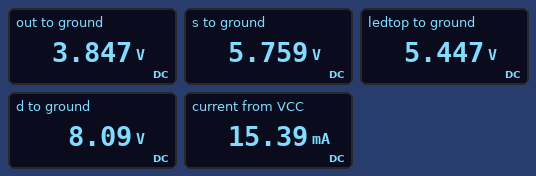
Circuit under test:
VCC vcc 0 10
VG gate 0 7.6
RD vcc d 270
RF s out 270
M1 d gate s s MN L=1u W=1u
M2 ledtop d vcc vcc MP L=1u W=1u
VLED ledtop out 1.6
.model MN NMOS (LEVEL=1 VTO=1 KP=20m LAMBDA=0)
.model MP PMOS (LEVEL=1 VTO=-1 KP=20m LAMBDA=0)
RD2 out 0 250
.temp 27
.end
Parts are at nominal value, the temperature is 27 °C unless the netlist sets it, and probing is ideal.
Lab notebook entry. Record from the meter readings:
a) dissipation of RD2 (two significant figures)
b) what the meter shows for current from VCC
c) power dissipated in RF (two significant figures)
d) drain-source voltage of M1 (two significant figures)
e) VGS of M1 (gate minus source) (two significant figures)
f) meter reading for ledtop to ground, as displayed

59 mW
15.39 mA
14 mW
2.3 V
1.8 V
5.447 V
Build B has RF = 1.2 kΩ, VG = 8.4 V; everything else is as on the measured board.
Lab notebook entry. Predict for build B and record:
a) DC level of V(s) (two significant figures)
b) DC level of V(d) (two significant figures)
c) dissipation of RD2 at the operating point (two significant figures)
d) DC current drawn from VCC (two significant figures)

6.7 V
8.8 V
6.4 mW
5.1 mA
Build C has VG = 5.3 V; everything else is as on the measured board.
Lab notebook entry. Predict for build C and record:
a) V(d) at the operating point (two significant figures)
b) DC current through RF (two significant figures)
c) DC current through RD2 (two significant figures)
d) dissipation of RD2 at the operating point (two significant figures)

8.5 V
5.6 mA
8.2 mA
17 mW
